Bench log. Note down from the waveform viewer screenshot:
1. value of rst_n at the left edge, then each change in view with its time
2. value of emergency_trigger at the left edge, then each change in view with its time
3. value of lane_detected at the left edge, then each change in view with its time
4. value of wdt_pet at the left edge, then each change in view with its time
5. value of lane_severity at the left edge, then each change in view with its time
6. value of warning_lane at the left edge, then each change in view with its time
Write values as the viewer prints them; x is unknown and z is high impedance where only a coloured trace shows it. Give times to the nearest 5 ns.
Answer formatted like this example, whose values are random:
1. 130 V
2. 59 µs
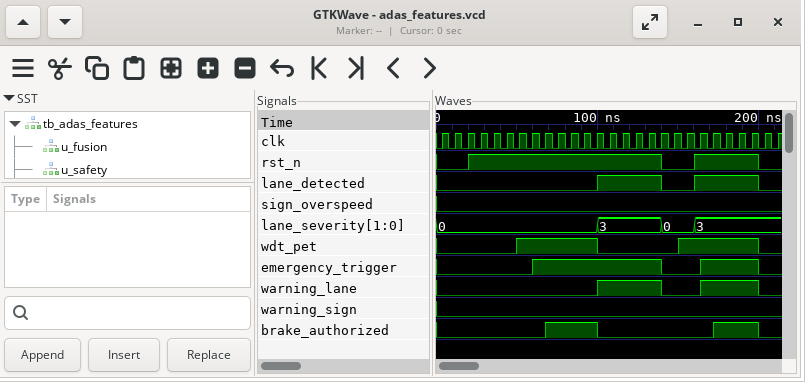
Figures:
1. 0, 1 at 20 ns, 0 at 140 ns, 1 at 160 ns, 0 at 200 ns
2. 0, 1 at 60 ns, 0 at 140 ns, 1 at 165 ns, 0 at 200 ns
3. 0, 1 at 100 ns, 0 at 140 ns, 1 at 160 ns, 0 at 200 ns
4. 0, 1 at 50 ns, 0 at 100 ns, 1 at 150 ns, 0 at 200 ns
5. 0, 3 at 100 ns, 0 at 140 ns, 3 at 160 ns
6. 0, 1 at 100 ns, 0 at 140 ns, 1 at 165 ns, 0 at 200 ns
